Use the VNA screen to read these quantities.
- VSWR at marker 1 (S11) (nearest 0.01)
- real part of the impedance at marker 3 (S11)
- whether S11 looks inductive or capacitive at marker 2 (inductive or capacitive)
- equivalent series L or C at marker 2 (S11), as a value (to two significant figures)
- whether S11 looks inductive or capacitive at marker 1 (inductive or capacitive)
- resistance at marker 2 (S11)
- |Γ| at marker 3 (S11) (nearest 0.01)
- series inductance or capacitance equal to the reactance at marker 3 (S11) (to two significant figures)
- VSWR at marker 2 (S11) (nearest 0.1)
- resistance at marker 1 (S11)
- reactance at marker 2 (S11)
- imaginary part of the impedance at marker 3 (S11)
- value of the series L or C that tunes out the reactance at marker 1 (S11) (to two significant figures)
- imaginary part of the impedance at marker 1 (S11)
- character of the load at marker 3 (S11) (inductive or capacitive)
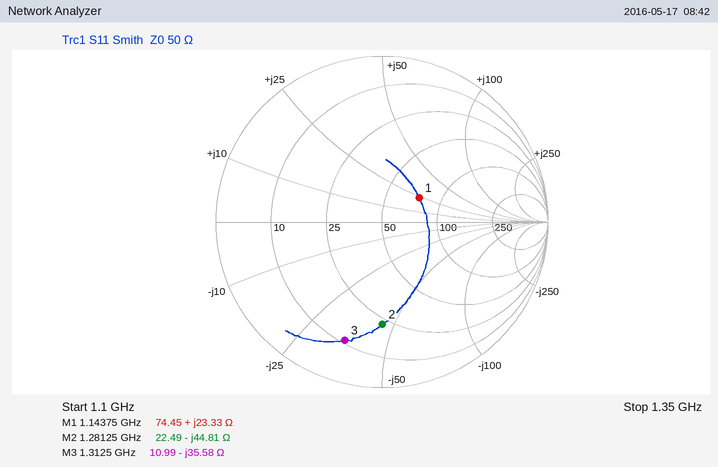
1.73
10.99 Ω
capacitive
2.8 pF
inductive
22.49 Ω
0.75
3.4 pF
4.2
74.45 Ω
-44.81 Ω
-35.58 Ω
6.0 pF
+23.33 Ω
capacitive
